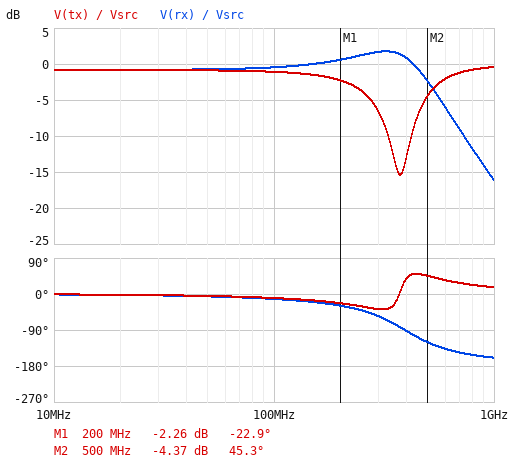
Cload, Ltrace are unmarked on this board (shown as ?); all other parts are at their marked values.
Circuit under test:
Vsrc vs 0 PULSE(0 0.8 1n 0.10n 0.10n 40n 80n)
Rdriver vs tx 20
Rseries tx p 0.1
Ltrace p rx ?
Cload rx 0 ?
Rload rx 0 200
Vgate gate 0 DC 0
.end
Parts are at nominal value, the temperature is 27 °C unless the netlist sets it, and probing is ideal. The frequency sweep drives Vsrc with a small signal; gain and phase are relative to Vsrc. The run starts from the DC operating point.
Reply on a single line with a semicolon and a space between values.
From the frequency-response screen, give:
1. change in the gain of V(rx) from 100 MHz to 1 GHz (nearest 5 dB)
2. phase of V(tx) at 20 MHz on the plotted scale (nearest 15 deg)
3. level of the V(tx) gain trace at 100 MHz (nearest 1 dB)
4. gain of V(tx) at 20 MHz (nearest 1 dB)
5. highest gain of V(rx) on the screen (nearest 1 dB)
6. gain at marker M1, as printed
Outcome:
-15 dB; 0 deg; -1 dB; -1 dB; 2 dB; -2.26 dB
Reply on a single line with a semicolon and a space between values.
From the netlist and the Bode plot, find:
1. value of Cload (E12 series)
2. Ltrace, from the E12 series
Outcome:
15 pF; 12 nH
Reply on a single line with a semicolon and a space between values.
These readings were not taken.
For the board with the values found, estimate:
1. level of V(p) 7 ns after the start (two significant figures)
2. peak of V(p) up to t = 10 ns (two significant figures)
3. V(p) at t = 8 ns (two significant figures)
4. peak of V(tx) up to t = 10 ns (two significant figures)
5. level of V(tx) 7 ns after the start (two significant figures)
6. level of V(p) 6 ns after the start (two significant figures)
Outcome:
730 mV; 800 mV; 730 mV; 800 mV; 730 mV; 730 mV
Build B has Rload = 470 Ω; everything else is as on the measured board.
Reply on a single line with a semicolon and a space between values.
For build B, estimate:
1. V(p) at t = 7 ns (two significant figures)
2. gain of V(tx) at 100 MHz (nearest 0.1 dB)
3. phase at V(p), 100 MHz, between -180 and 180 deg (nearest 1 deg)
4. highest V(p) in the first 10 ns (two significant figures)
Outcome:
770 mV; -0.6 dB; -11 deg; 860 mV
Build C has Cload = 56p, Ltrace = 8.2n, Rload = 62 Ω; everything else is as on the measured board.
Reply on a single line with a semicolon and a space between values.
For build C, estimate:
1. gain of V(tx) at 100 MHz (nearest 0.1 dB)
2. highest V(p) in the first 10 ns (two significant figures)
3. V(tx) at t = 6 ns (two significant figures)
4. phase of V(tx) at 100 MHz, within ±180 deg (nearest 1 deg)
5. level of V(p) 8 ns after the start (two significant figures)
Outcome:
-4.5 dB; 710 mV; 610 mV; -29 deg; 600 mV
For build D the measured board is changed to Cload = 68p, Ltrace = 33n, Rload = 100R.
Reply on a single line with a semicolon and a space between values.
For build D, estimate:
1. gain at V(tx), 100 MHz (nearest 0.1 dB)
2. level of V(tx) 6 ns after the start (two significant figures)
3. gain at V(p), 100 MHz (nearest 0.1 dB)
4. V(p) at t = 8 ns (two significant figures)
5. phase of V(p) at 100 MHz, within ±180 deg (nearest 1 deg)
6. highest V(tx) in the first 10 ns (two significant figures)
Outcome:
-13.3 dB; 640 mV; -13.4 dB; 710 mV; -12 deg; 780 mV
